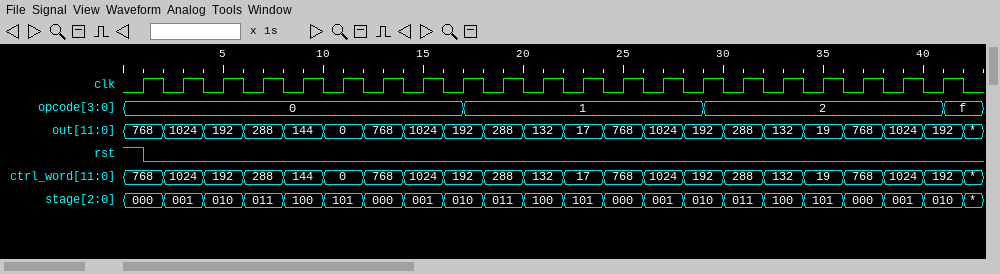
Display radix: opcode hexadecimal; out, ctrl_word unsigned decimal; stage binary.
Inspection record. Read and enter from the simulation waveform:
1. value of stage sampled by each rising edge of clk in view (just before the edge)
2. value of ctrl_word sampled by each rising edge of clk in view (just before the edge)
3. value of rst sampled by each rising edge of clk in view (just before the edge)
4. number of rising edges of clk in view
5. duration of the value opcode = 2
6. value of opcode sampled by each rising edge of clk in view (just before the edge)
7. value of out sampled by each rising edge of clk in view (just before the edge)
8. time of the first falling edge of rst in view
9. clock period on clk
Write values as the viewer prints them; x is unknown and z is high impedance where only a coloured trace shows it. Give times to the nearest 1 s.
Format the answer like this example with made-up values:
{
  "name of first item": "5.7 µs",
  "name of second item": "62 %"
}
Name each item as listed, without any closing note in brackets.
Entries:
{
  "value of stage sampled by each rising edge of clk in view": "000, 001, 010, 011, 100, 101, 000, 001, 010, 011, 100, 101, 000, 001, 010, 011, 100, 101, 000, 001, 010",
  "value of ctrl_word sampled by each rising edge of clk in view": "768, 1024, 192, 288, 144, 0, 768, 1024, 192, 288, 132, 17, 768, 1024, 192, 288, 132, 19, 768, 1024, 192",
  "value of rst sampled by each rising edge of clk in view": "1 0 0 0 0 0 0 0 0 0 0 0 0 0 0 0 0 0 0 0 0",
  "number of rising edges of clk in view": "21",
  "duration of the value opcode = 2": "12 s",
  "value of opcode sampled by each rising edge of clk in view": "0, 0, 0, 0, 0, 0, 0, 0, 0, 1, 1, 1, 1, 1, 1, 2, 2, 2, 2, 2, 2",
  "value of out sampled by each rising edge of clk in view": "768, 1024, 192, 288, 144, 0, 768, 1024, 192, 288, 132, 17, 768, 1024, 192, 288, 132, 19, 768, 1024, 192",
  "time of the first falling edge of rst in view": "1 s",
  "clock period on clk": "2 s"
}
